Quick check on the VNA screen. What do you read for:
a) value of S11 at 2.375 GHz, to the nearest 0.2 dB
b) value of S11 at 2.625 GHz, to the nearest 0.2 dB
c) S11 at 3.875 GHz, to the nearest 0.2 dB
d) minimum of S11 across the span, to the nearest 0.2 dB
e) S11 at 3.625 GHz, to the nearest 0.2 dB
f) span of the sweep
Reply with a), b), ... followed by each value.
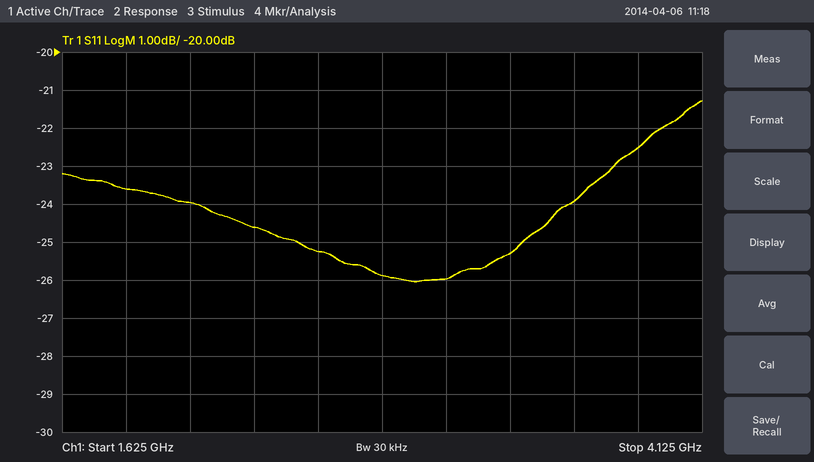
a) -24.6 dB
b) -25.2 dB
c) -22.6 dB
d) -26.0 dB
e) -24.0 dB
f) 2.5 GHz
